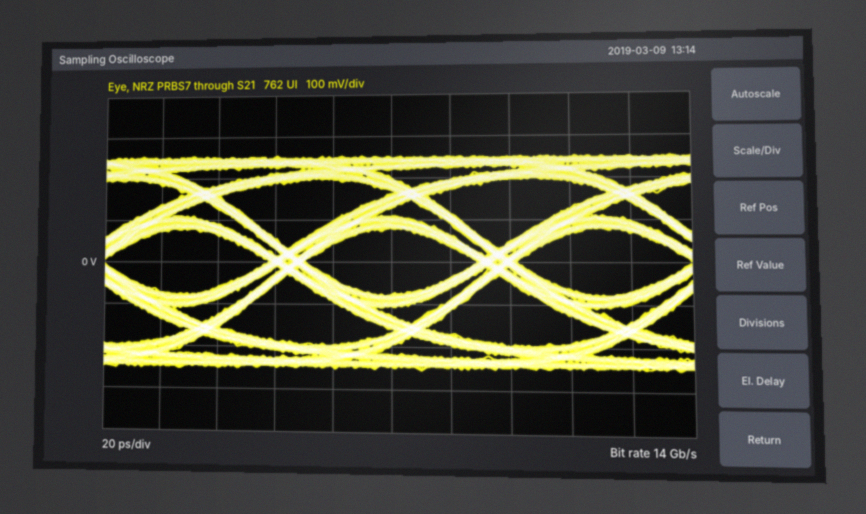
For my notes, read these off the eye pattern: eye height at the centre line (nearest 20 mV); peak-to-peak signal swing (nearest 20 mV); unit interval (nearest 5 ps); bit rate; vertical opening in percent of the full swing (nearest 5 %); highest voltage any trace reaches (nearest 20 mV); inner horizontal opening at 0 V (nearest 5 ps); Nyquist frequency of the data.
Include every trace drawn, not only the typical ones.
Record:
160 mV
500 mV
70 ps
14 Gb/s
30 %
260 mV
60 ps
7 GHz
